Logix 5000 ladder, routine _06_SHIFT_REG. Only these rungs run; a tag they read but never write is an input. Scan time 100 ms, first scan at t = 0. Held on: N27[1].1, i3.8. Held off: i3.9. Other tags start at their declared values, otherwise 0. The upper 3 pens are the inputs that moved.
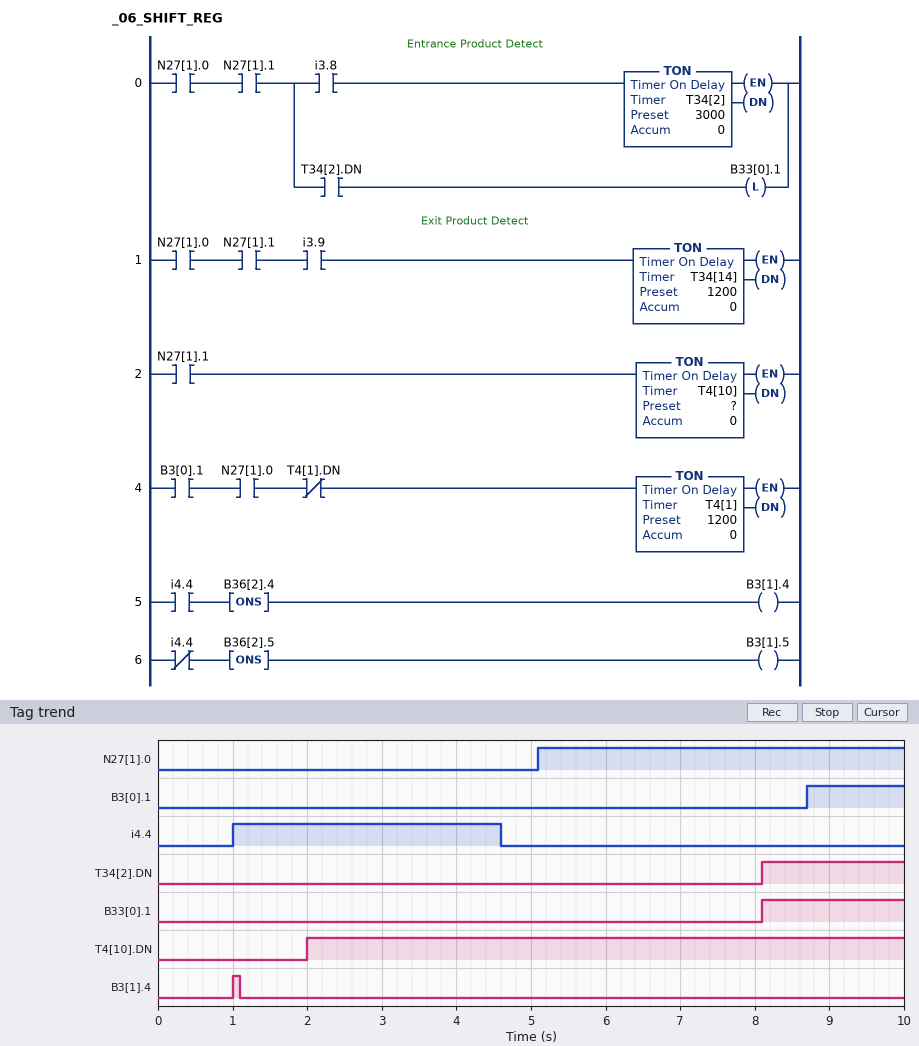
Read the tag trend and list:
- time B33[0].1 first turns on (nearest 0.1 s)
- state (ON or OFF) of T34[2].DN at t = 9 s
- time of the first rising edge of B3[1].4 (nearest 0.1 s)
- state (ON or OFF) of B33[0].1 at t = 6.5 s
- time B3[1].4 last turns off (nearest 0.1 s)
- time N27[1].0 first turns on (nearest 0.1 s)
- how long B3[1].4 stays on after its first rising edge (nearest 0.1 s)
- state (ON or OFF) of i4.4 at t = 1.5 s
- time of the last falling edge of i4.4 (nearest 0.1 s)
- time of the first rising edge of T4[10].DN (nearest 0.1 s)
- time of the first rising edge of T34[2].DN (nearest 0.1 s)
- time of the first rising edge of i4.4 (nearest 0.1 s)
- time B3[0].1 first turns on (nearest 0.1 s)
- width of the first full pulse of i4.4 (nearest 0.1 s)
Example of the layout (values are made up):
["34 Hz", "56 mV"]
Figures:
["8.1 s", "ON", "1.0 s", "OFF", "1.1 s", "5.1 s", "0.1 s", "ON", "4.6 s", "2.0 s", "8.1 s", "1.0 s", "8.7 s", "3.6 s"]
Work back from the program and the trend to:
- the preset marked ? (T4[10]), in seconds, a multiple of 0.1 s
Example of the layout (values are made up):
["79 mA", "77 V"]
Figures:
["2.0 s"]
